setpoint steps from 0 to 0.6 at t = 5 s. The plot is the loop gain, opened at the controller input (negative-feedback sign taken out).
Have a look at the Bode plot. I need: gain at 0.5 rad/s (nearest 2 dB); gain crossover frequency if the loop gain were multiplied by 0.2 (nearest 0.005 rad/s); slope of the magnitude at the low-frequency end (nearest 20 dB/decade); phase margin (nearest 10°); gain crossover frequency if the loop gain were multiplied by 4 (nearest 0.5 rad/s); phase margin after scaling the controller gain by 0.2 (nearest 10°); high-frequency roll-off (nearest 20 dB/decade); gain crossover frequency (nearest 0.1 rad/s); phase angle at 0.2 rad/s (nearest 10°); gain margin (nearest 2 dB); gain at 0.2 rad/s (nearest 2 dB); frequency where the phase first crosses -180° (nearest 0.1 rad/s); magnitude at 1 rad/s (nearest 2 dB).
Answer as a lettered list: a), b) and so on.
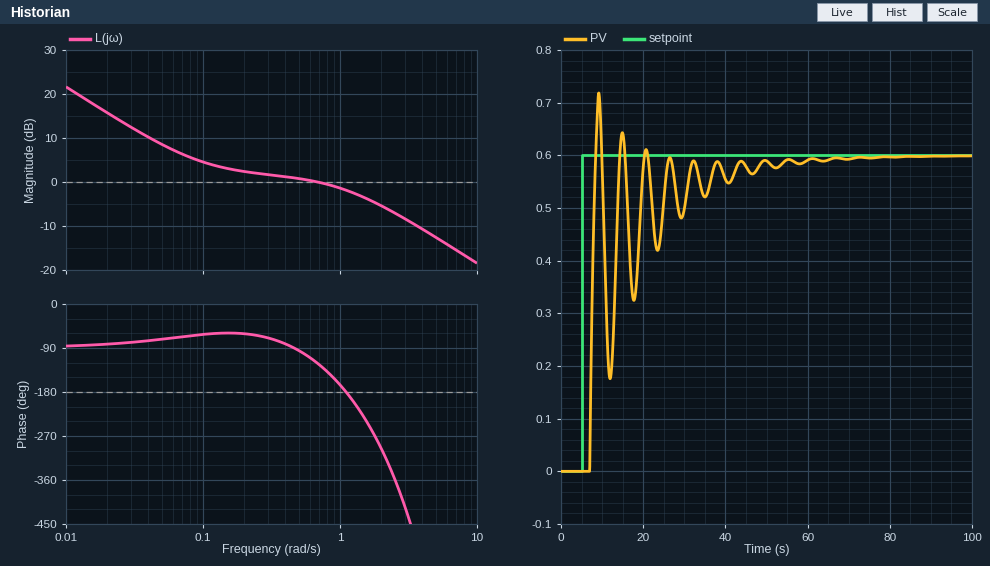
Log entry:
a) 0 dB
b) 0.025 rad/s
c) -20 dB/decade
d) 60°
e) 4.5 rad/s
f) 100°
g) -20 dB/decade
h) 0.7 rad/s
i) -60°
j) 2 dB
k) 2 dB
l) 1.1 rad/s
m) -2 dB
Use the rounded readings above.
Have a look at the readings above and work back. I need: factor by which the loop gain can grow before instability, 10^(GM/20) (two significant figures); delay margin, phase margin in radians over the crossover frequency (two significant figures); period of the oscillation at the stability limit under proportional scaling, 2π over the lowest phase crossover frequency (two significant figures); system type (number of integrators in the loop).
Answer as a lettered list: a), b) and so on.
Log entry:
a) 1.3
b) 1.5 s
c) 5.7 s
d) 1
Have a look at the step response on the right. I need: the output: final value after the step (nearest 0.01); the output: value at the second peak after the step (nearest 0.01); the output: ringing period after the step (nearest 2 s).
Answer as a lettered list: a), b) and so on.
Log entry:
a) 0.60
b) 0.64
c) 6 s
